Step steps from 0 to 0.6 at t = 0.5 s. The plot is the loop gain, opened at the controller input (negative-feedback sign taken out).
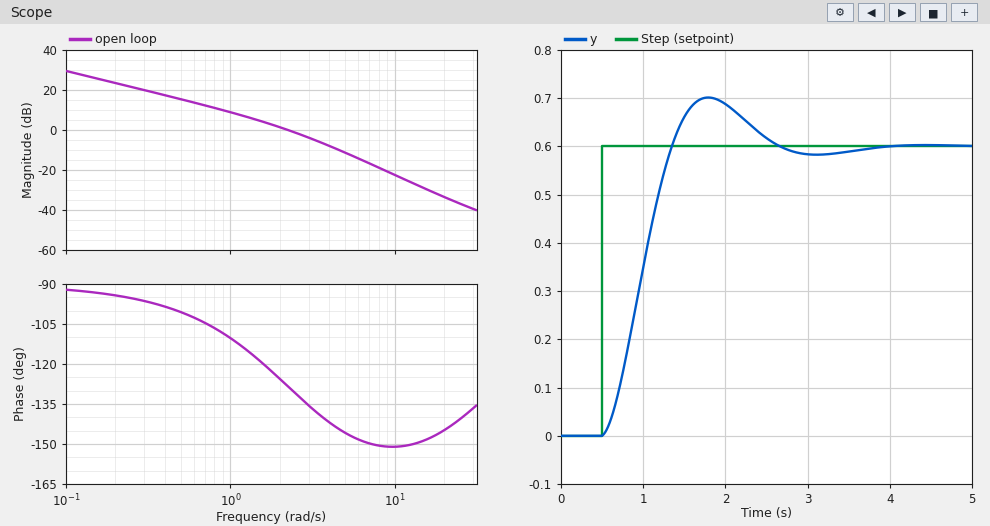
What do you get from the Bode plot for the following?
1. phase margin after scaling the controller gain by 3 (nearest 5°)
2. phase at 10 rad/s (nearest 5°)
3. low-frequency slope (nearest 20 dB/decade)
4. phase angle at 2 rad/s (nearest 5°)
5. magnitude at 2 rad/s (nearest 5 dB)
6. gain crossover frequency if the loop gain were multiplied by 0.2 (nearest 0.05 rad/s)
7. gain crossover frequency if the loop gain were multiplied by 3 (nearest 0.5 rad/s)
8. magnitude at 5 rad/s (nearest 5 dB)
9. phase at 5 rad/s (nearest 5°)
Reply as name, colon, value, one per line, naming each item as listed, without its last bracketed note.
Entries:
phase margin after scaling the controller gain by 3: 35°
phase at 10 rad/s: -150°
low-frequency slope: -20 dB/decade
phase angle at 2 rad/s: -125°
magnitude at 2 rad/s: 0 dB
gain crossover frequency if the loop gain were multiplied by 0.2: 0.60 rad/s
gain crossover frequency if the loop gain were multiplied by 3: 4.5 rad/s
magnitude at 5 rad/s: -10 dB
phase at 5 rad/s: -145°
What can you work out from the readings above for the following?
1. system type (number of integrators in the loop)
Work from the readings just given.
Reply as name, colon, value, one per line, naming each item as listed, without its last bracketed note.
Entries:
system type: 1
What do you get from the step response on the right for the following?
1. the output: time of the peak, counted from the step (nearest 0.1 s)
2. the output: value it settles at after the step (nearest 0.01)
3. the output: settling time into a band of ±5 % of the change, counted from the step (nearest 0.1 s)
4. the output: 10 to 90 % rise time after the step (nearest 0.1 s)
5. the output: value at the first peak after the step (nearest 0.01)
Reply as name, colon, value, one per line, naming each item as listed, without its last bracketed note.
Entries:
the output: time of the peak, counted from the step: 1.3 s
the output: value it settles at after the step: 0.60
the output: settling time into a band of ±5 % of the change, counted from the step: 1.9 s
the output: 10 to 90 % rise time after the step: 0.6 s
the output: value at the first peak after the step: 0.70
